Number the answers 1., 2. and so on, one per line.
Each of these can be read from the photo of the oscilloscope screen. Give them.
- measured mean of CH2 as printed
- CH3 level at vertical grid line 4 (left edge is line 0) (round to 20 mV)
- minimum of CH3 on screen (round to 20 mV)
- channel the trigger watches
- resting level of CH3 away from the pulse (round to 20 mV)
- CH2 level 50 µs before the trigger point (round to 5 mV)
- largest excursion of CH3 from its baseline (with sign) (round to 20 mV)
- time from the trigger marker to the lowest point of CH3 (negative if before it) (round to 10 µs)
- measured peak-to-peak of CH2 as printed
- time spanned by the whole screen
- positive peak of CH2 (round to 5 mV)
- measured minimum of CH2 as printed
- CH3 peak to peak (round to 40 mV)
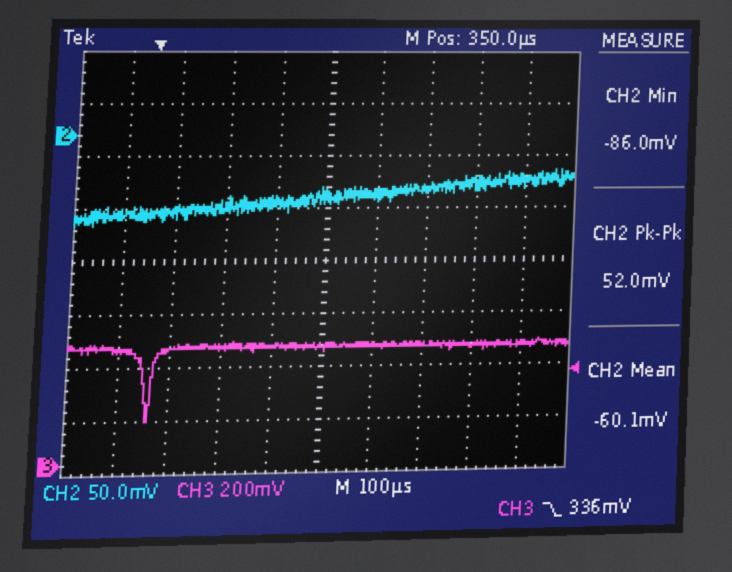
1. -60.1 mV
2. 440 mV
3. 160 mV
4. CH3
5. 440 mV
6. -75 mV
7. -280 mV
8. +10 µs
9. 52.0 mV
10. 1 ms
11. -35 mV
12. -86.0 mV
13. 280 mV
